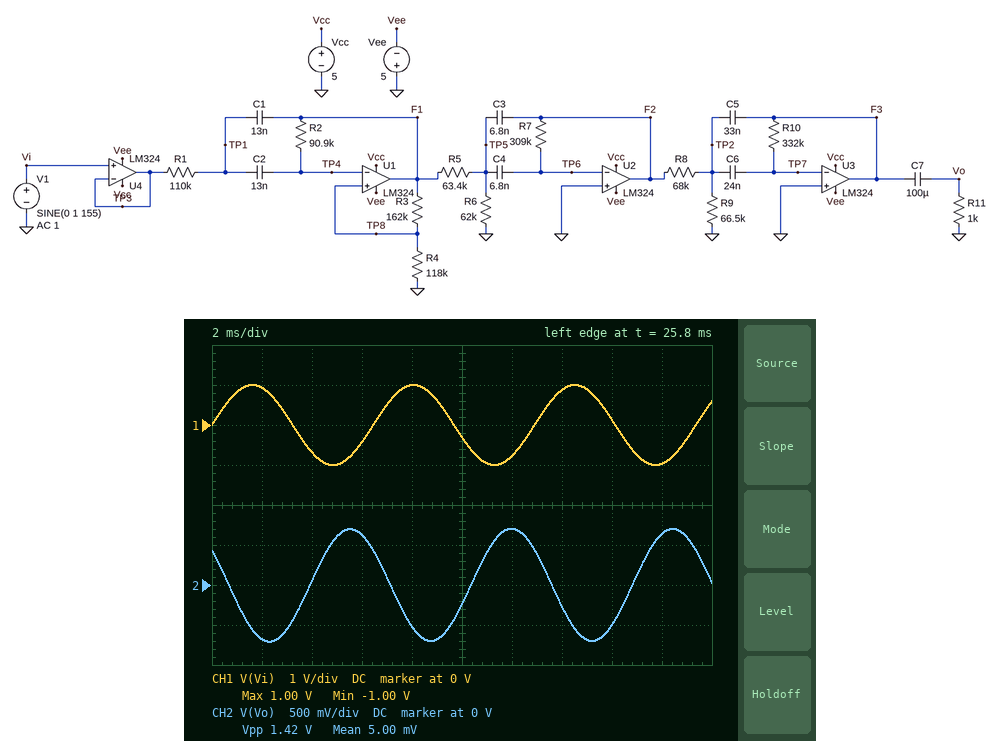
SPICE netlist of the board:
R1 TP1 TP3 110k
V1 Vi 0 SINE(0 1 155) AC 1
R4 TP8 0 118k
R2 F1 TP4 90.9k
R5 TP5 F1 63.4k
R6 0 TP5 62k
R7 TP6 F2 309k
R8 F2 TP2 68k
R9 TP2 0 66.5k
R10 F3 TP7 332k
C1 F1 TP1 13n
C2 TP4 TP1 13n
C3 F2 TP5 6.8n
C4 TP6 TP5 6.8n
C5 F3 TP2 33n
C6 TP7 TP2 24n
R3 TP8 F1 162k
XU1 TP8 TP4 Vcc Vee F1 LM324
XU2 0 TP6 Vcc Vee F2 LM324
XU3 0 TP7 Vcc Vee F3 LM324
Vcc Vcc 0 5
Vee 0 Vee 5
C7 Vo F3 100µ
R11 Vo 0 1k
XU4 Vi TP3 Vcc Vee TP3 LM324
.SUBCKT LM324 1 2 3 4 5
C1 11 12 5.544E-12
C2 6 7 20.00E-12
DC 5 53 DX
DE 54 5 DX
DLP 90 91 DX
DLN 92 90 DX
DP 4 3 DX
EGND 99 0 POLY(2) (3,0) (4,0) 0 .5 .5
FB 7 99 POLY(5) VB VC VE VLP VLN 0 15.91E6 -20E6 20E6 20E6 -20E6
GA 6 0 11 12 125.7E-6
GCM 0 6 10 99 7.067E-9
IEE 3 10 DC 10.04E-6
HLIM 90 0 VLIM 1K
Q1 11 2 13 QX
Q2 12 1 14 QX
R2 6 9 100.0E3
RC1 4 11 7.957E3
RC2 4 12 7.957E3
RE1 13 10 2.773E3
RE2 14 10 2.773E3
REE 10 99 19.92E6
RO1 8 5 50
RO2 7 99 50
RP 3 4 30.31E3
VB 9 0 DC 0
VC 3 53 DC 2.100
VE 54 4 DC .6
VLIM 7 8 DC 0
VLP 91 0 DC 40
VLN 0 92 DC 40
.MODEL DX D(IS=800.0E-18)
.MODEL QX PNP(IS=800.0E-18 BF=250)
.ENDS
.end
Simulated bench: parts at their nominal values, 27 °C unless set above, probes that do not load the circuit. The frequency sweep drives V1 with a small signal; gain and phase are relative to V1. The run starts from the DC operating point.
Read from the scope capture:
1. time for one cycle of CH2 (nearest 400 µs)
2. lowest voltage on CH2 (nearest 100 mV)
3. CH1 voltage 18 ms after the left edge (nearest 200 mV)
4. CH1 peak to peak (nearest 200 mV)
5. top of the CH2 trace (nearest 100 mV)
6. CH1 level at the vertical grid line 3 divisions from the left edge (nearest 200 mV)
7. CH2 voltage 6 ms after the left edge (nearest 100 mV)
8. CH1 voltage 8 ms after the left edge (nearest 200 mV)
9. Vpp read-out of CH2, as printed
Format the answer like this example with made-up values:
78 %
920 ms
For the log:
6.4 ms
-700 mV
-1.0 V
2.0 V
700 mV
-400 mV
600 mV
1.0 V
1.42 V
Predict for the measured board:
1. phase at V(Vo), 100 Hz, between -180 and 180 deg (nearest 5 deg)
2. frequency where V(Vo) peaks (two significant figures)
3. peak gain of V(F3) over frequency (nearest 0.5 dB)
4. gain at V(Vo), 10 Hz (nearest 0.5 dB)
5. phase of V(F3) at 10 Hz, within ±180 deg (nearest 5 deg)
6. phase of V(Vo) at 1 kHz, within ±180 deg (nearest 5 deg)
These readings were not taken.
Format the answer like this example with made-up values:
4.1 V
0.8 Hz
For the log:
-155 deg
170 Hz
-3.0 dB
-53.5 dB
75 deg
-70 deg
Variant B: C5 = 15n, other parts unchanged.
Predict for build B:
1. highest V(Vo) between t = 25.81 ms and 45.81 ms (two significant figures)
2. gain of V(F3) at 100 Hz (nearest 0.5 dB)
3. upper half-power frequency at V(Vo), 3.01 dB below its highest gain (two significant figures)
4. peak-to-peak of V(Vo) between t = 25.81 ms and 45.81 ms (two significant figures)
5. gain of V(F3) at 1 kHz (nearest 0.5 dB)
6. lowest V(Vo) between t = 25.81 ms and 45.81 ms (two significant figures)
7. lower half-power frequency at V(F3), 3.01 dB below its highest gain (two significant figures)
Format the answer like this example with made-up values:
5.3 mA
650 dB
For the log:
1.7 V
5.0 dB
240 Hz
3.5 V
-38.5 dB
-1.7 V
74 Hz
